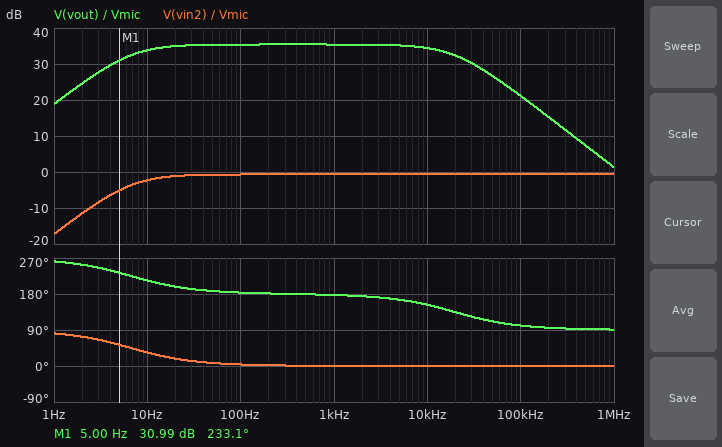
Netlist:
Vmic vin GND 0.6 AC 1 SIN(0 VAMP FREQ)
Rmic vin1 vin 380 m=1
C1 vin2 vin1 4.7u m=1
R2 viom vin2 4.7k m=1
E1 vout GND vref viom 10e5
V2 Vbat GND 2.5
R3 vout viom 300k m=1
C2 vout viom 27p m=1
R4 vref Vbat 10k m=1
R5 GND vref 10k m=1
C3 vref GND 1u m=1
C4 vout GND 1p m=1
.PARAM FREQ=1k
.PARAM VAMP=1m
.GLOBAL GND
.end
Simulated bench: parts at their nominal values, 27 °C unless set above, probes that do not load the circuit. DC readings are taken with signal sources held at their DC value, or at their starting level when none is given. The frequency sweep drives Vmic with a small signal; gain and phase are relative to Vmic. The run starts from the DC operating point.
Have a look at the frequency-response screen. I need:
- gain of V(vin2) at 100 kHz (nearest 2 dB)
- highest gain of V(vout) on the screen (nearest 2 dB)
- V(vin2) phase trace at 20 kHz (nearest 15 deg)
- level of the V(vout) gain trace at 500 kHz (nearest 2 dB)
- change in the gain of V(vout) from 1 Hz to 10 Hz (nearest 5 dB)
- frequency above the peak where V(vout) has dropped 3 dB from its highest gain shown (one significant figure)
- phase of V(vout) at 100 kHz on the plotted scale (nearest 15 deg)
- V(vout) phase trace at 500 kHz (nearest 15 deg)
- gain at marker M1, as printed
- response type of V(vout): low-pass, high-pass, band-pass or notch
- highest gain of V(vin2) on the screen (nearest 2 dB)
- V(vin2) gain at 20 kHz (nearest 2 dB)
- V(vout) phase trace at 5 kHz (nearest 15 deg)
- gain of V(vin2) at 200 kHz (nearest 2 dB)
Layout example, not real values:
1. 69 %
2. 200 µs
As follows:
1. 0 dB
2. 36 dB
3. 0 deg
4. 8 dB
5. 15 dB
6. 20 kHz
7. 105 deg
8. 90 deg
9. 30.99 dB
10. band-pass
11. 0 dB
12. 0 dB
13. 165 deg
14. 0 dB
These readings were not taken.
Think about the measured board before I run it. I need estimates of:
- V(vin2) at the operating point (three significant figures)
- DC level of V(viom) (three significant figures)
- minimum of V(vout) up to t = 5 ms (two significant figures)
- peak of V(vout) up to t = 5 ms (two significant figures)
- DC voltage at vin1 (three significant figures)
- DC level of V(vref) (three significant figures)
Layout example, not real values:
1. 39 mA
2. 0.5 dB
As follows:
1. 1.25 V
2. 1.25 V
3. 1.2 V
4. 1.3 V
5. 600 mV
6. 1.25 V
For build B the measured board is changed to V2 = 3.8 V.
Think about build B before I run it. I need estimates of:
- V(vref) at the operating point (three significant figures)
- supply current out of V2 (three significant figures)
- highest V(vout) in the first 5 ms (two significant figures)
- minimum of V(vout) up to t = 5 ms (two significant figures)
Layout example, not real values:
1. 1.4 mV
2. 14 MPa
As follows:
1. 1.90 V
2. 190 µA
3. 2.0 V
4. 1.8 V
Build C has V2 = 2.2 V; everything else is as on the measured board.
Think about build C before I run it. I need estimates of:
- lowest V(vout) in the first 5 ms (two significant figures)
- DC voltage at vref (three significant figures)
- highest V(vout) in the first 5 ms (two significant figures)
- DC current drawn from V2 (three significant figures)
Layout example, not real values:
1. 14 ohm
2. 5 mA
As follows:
1. 1.0 V
2. 1.10 V
3. 1.2 V
4. 110 µA
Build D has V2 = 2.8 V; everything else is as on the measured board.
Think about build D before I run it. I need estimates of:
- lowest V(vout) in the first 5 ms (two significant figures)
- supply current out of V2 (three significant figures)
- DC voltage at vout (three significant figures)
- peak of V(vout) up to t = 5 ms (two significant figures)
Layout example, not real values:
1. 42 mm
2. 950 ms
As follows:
1. 1.3 V
2. 140 µA
3. 1.40 V
4. 1.5 V
